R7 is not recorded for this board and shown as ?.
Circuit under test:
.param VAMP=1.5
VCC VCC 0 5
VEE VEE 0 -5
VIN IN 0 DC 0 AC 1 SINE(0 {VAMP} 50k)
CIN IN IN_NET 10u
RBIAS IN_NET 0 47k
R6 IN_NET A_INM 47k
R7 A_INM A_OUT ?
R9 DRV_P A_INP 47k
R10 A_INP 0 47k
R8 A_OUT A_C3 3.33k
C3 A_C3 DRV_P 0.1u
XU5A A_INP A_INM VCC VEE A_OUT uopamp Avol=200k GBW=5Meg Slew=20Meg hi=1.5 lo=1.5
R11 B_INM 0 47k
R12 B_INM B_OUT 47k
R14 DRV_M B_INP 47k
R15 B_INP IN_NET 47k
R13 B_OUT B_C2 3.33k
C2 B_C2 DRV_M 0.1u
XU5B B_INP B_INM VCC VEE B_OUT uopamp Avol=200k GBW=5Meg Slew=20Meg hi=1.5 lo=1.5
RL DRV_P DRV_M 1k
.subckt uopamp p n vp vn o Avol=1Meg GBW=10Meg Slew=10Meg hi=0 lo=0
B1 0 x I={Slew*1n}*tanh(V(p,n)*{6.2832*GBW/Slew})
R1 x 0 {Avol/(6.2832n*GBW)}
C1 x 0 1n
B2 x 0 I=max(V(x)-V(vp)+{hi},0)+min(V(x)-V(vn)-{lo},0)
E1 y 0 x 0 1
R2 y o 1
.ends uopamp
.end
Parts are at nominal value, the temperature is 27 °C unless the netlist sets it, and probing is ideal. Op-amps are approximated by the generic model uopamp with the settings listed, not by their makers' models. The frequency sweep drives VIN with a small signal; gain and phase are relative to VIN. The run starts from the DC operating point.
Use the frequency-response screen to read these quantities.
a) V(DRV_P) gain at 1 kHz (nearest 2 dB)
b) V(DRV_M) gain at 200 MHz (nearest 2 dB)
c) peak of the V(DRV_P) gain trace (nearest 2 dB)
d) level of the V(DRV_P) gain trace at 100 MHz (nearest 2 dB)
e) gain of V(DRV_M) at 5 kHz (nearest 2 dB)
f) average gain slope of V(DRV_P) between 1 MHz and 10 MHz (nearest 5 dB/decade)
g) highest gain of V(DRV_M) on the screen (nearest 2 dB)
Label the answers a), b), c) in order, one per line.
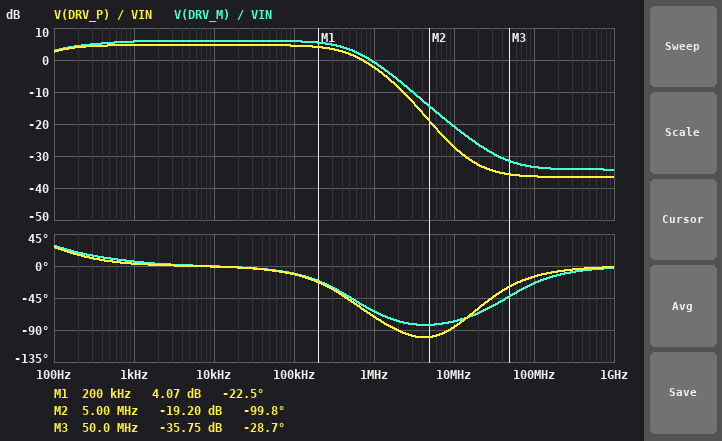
a) 4 dB
b) -34 dB
c) 4 dB
d) -36 dB
e) 6 dB
f) -25 dB/decade
g) 6 dB
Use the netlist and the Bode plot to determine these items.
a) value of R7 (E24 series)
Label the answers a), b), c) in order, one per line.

a) 16 kΩ
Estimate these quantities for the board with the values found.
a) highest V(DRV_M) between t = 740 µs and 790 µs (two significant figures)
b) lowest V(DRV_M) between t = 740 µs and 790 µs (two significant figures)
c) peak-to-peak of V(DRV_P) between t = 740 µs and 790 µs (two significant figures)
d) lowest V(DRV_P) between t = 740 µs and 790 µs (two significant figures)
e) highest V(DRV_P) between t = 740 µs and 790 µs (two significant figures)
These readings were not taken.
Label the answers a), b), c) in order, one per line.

a) 2.3 V
b) -2.3 V
c) 4.0 V
d) -2.0 V
e) 2.0 V
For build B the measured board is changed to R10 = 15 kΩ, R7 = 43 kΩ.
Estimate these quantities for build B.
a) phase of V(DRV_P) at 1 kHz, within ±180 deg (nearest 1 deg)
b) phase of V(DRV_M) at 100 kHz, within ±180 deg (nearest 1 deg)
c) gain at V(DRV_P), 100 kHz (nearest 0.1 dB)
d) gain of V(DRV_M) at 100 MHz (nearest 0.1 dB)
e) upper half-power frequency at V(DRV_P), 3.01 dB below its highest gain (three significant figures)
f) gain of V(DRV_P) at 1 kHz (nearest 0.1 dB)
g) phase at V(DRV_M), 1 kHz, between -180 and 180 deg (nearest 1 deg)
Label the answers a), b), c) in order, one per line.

a) -5 deg
b) -7 deg
c) -15.2 dB
d) -34.1 dB
e) 89.5 Hz
f) -15.0 dB
g) 13 deg
